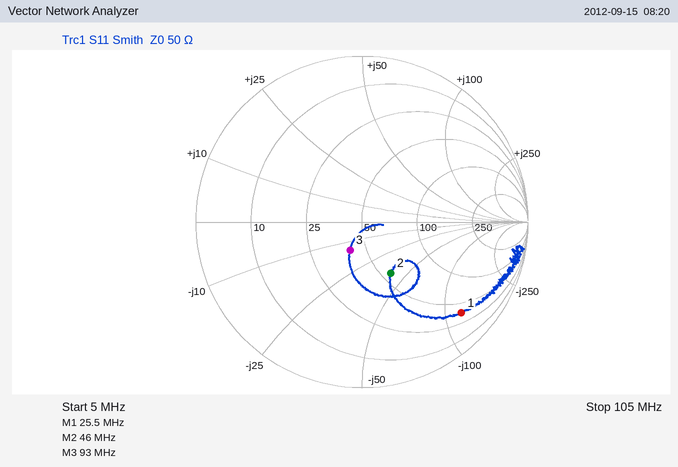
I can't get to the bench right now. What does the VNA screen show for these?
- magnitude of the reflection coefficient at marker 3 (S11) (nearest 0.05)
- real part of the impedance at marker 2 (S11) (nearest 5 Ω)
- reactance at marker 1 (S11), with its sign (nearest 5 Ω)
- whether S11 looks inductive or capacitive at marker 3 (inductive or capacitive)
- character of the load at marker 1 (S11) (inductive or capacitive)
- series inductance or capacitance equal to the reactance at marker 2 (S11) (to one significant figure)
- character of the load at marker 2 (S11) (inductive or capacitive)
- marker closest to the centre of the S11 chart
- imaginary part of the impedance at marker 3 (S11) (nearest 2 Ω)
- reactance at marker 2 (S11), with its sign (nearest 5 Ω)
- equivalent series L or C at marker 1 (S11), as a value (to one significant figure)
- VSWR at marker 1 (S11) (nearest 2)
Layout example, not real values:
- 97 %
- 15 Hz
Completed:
- 0.20
- 55 Ω
- -120 Ω
- capacitive
- capacitive
- 90 pF
- capacitive
- marker 3
- -14 Ω
- -40 Ω
- 50 pF
- 10
